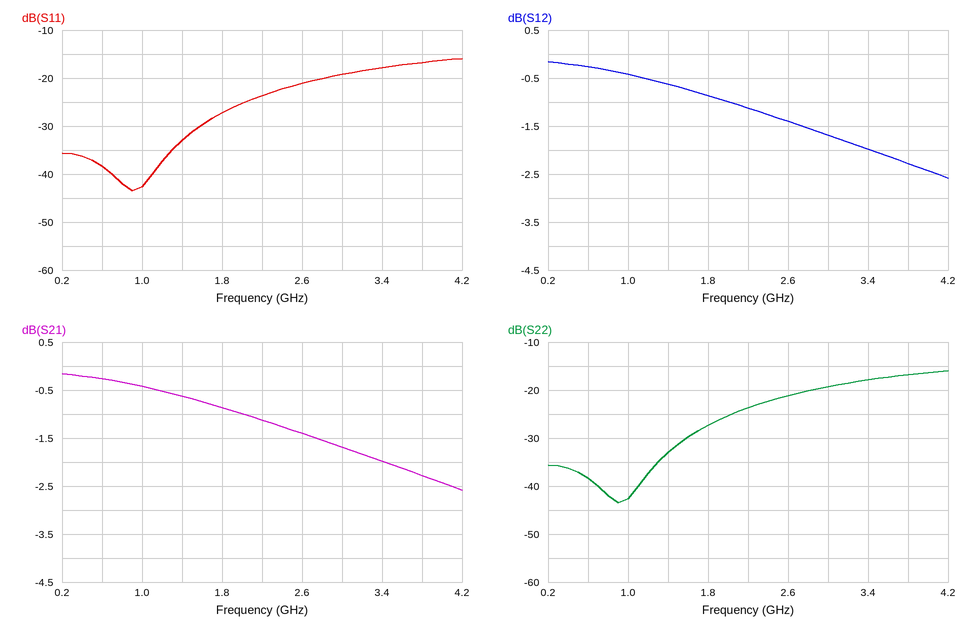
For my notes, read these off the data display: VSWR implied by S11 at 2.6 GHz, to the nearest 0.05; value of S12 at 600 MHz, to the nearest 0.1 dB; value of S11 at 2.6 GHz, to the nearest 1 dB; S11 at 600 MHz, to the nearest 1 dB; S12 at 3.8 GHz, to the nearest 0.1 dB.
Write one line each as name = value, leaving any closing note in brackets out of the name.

VSWR implied by S11 at 2.6 GHz, to the nearest 0.05 = 1.20
value of S12 at 600 MHz, to the nearest 0.1 dB = -0.3 dB
value of S11 at 2.6 GHz, to the nearest 1 dB = -21 dB
S11 at 600 MHz, to the nearest 1 dB = -38 dB
S12 at 3.8 GHz, to the nearest 0.1 dB = -2.3 dB
